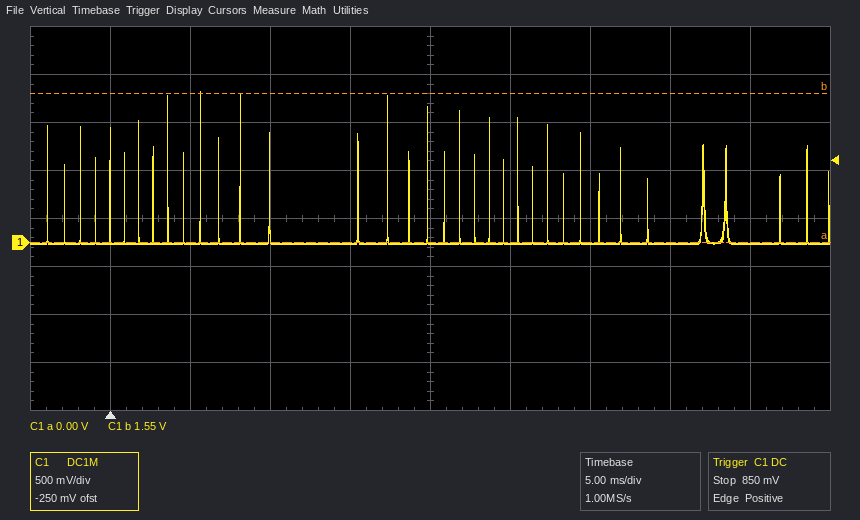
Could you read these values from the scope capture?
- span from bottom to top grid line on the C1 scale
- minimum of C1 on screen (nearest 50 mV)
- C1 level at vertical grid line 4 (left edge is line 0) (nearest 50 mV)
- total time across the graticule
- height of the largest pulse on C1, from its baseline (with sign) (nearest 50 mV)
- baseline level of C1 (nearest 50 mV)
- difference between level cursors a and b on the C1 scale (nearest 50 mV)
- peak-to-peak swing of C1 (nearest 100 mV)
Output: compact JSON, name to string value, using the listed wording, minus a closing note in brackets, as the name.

{"span from bottom to top grid line on the C1 scale": "4 V", "minimum of C1 on screen": "0 mV", "C1 level at vertical grid line 4 (left edge is line 0)": "0 mV", "total time across the graticule": "50 ms", "height of the largest pulse on C1, from its baseline (with sign)": "+1.60 V", "baseline level of C1": "0 mV", "difference between level cursors a and b on the C1 scale": "1.55 V", "peak-to-peak swing of C1": "1.60 V"}
